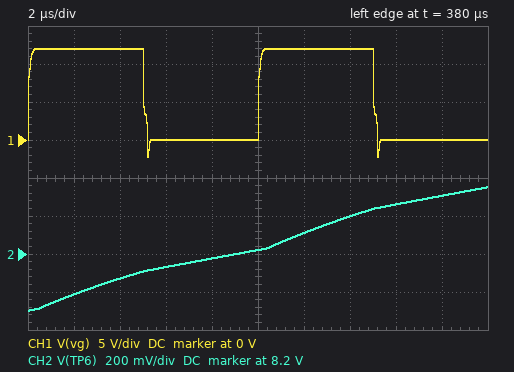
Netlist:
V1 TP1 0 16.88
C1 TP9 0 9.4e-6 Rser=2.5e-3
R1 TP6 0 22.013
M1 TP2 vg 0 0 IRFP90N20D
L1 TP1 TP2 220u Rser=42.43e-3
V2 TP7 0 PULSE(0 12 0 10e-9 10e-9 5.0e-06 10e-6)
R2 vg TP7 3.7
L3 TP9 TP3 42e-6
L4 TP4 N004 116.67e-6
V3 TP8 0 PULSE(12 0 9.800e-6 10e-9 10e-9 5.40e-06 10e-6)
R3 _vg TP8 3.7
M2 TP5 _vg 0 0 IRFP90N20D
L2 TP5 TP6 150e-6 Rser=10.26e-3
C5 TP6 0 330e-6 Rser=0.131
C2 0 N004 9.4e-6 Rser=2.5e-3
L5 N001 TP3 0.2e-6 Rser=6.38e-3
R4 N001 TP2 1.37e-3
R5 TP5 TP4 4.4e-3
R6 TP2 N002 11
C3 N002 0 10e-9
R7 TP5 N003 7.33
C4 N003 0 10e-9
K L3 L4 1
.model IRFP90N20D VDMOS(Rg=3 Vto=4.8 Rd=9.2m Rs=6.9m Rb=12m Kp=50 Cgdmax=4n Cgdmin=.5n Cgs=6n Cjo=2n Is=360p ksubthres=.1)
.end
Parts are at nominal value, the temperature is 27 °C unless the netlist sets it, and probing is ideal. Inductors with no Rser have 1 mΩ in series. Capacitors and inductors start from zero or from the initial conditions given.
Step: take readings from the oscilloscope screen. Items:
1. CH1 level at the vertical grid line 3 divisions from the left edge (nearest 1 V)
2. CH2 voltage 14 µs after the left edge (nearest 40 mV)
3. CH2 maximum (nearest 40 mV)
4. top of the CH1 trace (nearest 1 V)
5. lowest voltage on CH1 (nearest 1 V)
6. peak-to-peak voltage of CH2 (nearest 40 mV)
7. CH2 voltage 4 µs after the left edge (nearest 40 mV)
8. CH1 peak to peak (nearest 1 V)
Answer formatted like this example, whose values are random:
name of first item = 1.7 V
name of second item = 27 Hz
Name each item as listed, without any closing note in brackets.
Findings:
CH1 level at the vertical grid line 3 divisions from the left edge = 0 V
CH2 voltage 14 µs after the left edge = 8.40 V
CH2 maximum = 8.56 V
top of the CH1 trace = 12 V
lowest voltage on CH1 = -2 V
peak-to-peak voltage of CH2 = 640 mV
CH2 voltage 4 µs after the left edge = 8.08 V
CH1 peak to peak = 14 V
